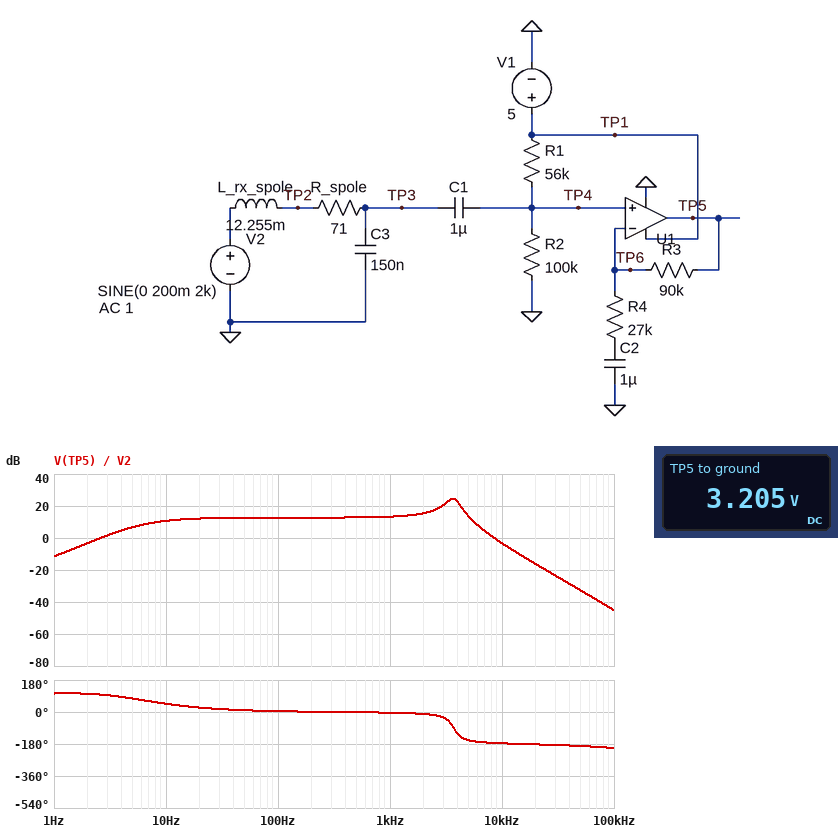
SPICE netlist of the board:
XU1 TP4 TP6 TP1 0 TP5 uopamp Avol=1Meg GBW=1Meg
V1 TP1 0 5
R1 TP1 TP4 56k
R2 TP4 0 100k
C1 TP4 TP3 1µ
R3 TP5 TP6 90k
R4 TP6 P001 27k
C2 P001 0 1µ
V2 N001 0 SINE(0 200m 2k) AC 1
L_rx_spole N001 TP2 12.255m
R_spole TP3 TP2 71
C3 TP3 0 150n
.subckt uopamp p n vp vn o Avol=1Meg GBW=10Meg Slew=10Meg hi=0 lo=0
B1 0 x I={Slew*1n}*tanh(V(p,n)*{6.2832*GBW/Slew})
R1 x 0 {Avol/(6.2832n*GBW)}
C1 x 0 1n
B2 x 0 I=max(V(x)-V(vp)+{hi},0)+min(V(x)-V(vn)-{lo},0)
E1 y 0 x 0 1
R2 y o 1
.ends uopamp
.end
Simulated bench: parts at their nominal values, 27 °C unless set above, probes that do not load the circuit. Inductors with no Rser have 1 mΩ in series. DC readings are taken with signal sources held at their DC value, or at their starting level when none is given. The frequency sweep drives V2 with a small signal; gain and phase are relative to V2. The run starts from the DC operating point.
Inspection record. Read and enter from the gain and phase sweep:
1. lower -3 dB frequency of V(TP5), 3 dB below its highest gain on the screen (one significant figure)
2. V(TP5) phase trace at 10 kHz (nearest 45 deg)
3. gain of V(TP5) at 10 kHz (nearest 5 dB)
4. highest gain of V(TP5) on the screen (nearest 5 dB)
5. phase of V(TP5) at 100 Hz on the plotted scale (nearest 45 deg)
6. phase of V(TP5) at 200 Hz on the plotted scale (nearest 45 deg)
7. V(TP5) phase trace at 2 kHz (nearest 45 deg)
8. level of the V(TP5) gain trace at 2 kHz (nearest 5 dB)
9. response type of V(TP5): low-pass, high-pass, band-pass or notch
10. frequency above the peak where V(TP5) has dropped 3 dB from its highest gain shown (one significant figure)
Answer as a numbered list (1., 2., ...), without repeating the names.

1. 3 kHz
2. -180 deg
3. -5 dB
4. 25 dB
5. 0 deg
6. 0 deg
7. 0 deg
8. 15 dB
9. band-pass
10. 4 kHz
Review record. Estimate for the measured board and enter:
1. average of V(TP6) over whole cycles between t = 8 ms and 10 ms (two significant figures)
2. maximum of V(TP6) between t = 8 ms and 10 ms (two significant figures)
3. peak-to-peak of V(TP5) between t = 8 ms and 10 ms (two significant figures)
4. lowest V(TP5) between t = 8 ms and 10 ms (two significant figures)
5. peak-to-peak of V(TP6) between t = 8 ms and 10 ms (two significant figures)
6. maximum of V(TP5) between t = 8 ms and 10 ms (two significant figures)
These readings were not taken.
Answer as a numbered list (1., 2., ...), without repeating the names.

1. 3.2 V
2. 3.5 V
3. 2.4 V
4. 2.0 V
5. 550 mV
6. 4.4 V
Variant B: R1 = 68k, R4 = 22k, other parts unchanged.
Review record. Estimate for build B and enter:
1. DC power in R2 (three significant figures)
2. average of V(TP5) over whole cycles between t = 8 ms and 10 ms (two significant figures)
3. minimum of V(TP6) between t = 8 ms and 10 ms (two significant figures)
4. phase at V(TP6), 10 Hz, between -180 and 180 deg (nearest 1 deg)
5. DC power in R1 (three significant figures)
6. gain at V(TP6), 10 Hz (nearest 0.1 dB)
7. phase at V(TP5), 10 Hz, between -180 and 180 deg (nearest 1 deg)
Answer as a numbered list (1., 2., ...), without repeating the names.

1. 88.6 µW
2. 3.0 V
3. 2.7 V
4. 21 deg
5. 60.2 µW
6. -0.6 dB
7. 49 deg
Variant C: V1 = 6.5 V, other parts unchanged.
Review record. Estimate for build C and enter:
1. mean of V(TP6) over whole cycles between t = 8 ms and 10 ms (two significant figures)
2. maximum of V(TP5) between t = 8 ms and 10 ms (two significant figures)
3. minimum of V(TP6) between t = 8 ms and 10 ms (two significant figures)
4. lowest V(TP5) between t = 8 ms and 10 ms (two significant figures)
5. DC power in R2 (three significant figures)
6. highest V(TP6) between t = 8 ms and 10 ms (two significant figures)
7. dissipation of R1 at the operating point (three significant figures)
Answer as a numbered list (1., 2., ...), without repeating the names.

1. 4.2 V
2. 5.4 V
3. 3.9 V
4. 3.0 V
5. 174 µW
6. 4.4 V
7. 97.2 µW
